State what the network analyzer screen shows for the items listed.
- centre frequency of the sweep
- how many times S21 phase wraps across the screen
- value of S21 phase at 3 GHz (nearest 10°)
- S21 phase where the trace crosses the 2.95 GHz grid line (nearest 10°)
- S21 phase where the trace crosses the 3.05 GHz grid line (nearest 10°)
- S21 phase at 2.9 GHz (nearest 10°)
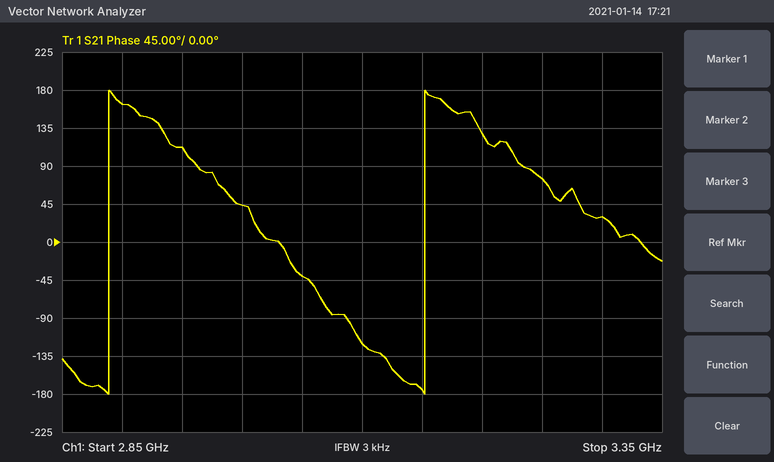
3.1 GHz
2
40°
110°
-40°
160°
